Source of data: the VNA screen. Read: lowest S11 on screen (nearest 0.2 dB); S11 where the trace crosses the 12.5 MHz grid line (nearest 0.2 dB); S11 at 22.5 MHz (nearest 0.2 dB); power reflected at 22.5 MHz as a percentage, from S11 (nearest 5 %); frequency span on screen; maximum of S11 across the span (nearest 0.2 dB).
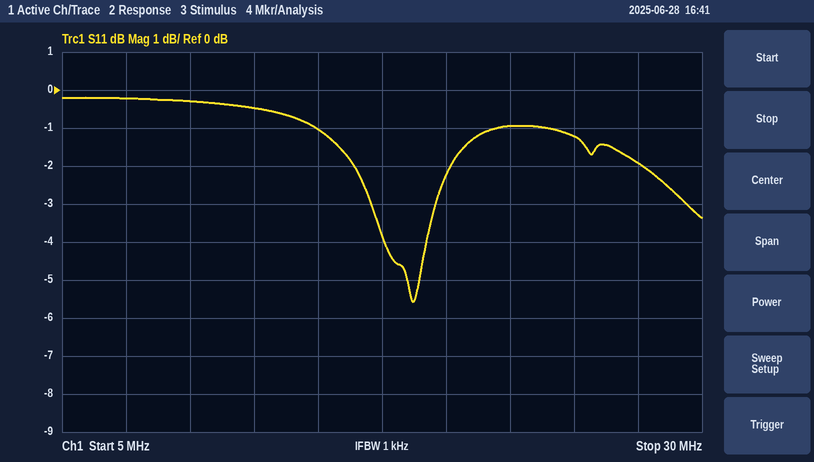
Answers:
-5.6 dB
-0.4 dB
-1.0 dB
80 %
25 MHz
-0.2 dB
